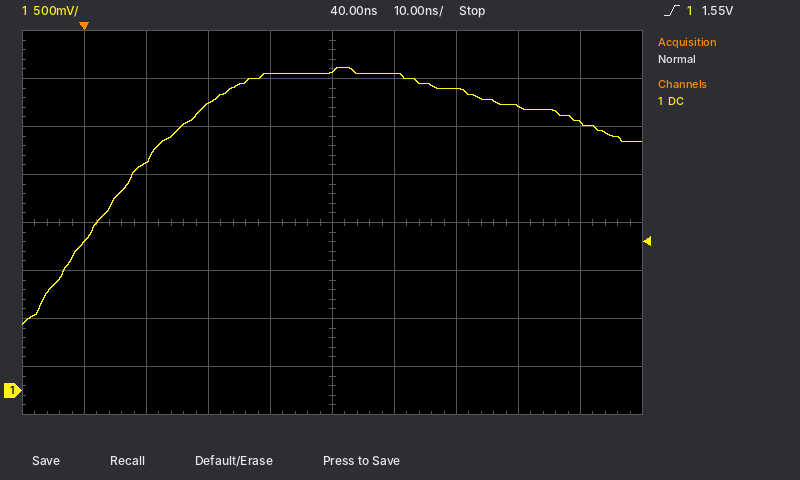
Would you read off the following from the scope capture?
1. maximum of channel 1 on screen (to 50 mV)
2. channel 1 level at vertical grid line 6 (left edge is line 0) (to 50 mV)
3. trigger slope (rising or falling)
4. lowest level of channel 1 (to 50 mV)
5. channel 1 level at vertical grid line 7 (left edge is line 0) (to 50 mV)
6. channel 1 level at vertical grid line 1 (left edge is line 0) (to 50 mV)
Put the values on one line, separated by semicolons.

3.35 V; 3.30 V; rising; 700 mV; 3.15 V; 1.55 V
